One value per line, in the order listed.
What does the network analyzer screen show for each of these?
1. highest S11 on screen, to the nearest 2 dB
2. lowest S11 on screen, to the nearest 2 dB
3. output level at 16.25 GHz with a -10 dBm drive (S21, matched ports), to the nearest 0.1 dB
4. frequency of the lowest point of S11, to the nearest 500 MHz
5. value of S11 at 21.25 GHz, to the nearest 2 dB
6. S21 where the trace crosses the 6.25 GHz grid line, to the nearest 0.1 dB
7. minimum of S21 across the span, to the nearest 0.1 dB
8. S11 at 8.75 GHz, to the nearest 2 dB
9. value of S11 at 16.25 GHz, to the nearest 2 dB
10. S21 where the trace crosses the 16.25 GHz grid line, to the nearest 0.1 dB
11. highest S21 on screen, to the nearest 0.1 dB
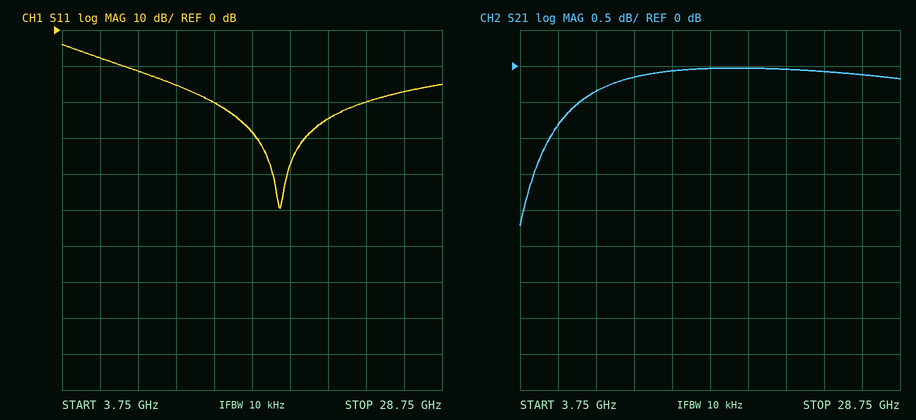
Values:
-4 dB
-50 dB
-10.0 dBm
18.0 GHz
-24 dB
-0.8 dB
-2.2 dB
-12 dB
-28 dB
0.0 dB
0.0 dB
